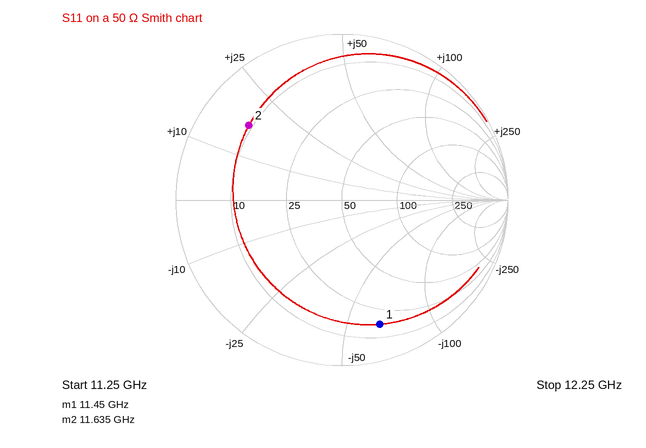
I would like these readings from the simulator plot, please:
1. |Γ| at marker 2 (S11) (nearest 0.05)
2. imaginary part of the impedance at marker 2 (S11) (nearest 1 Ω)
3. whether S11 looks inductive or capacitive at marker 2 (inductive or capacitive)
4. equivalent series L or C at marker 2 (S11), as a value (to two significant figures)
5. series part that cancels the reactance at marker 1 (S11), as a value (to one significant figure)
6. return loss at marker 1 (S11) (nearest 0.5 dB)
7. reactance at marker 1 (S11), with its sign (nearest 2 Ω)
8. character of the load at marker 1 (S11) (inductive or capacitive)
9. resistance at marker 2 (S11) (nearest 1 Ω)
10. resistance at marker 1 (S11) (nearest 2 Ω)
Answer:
0.70
+17 Ω
inductive
230 pH
900 pH
2.0 dB
-64 Ω
capacitive
9 Ω
16 Ω
